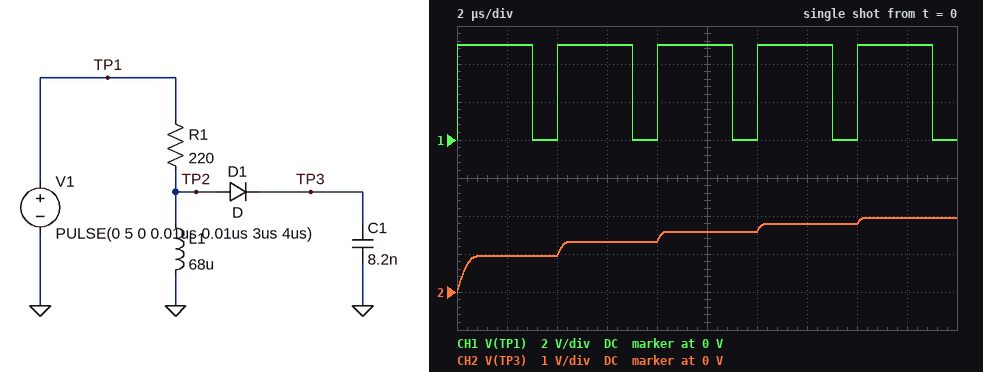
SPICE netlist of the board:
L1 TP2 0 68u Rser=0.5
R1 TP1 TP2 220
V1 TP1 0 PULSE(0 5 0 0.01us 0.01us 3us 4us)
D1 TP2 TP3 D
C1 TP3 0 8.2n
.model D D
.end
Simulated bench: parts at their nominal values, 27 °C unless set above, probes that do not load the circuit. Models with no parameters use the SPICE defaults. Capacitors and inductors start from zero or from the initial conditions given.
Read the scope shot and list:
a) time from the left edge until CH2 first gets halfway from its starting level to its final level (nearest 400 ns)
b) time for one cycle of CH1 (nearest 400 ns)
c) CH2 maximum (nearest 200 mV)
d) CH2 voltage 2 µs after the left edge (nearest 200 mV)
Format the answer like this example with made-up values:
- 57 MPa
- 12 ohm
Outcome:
- 4.0 µs
- 4.0 µs
- 2.0 V
- 1.0 V
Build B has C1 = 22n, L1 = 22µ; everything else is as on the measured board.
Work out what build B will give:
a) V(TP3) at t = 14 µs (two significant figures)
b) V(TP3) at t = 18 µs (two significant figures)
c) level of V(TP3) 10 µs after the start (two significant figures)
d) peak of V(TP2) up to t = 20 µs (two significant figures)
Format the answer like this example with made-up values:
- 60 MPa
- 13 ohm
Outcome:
- 610 mV
- 710 mV
- 500 mV
- 1.4 V
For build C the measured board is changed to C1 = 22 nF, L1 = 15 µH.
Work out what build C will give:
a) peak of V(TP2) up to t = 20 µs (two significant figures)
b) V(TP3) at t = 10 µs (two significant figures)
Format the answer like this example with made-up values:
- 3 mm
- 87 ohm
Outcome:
- 1.2 V
- 380 mV
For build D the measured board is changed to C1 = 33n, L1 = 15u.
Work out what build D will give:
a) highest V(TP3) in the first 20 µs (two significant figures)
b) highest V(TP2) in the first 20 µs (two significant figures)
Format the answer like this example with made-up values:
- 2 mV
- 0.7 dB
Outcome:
- 410 mV
- 1.1 V
